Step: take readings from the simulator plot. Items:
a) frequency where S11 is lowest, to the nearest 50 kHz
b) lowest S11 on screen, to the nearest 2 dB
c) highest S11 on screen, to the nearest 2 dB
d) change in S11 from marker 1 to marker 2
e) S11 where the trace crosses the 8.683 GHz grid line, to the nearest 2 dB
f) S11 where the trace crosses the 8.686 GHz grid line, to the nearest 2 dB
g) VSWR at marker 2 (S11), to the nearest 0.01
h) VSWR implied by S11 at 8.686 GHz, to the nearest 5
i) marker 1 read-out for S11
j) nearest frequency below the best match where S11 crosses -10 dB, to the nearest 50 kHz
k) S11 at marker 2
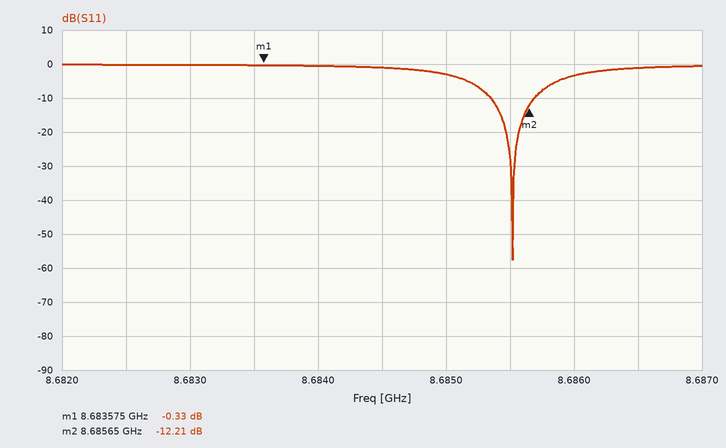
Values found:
8.68550 GHz
-58 dB
0 dB
-11.88 dB
0 dB
-4 dB
1.65
5
-0.33 dB
8.68535 GHz
-12.21 dB
